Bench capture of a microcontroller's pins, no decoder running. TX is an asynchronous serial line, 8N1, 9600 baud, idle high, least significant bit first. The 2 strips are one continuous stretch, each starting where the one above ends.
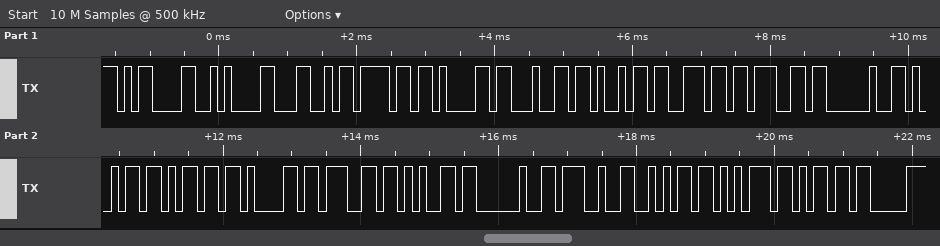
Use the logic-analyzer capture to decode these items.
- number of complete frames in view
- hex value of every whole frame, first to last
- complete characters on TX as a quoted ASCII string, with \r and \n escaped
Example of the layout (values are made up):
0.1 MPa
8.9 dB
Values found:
20
0D 0A 4C 6F 61 64 69 6E 67 20 69 6D 61 67 65 20 27 6A 75 6D
"\r\nLoading image 'jum"
